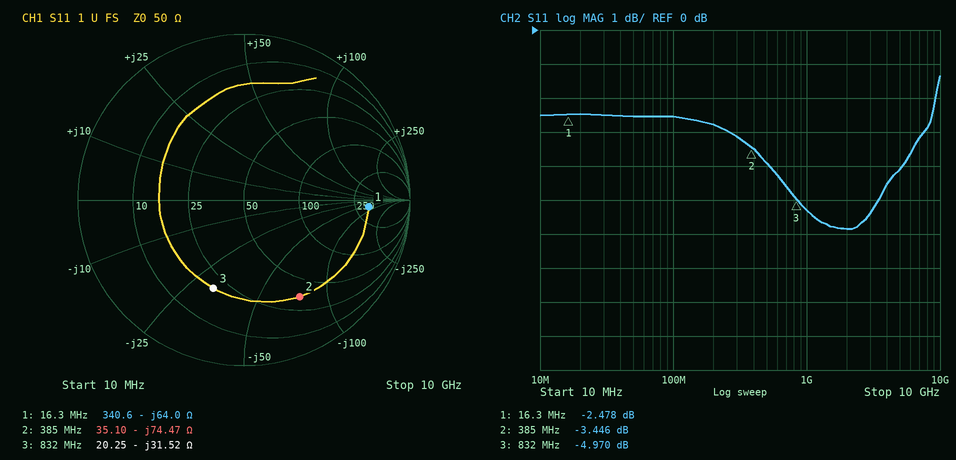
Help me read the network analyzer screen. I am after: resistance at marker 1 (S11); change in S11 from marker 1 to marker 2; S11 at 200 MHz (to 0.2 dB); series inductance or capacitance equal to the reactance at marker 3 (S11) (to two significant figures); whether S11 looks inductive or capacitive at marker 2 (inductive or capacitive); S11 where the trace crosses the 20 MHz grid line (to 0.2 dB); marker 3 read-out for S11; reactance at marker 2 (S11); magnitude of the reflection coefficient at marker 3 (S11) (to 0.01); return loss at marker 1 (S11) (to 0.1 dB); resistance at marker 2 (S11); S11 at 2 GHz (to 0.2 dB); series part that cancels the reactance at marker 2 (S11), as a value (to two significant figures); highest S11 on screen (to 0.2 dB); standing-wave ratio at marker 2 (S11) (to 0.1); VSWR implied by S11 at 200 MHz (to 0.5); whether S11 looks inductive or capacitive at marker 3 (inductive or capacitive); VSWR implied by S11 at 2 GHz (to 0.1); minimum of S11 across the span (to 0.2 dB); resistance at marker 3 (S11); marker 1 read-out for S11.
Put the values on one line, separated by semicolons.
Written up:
340.6 Ω; -0.968 dB; -2.8 dB; 6.1 pF; capacitive; -2.4 dB; -4.970 dB; -74.47 Ω; 0.56; 2.5 dB; 35.10 Ω; -5.8 dB; 31 nH; -1.4 dB; 5.1; 6.5; capacitive; 3.1; -5.8 dB; 20.25 Ω; -2.478 dB
